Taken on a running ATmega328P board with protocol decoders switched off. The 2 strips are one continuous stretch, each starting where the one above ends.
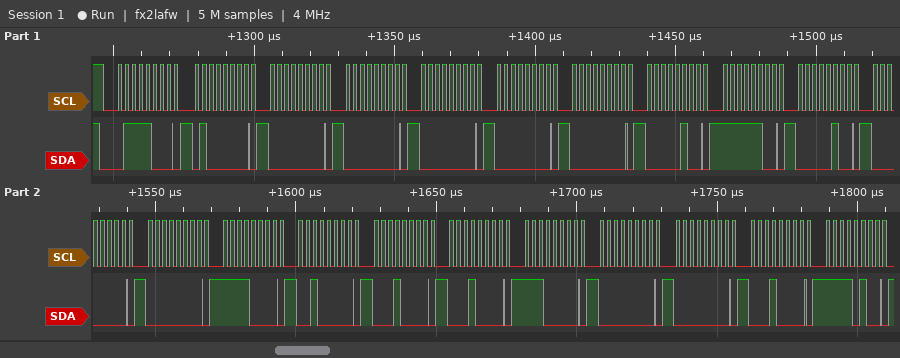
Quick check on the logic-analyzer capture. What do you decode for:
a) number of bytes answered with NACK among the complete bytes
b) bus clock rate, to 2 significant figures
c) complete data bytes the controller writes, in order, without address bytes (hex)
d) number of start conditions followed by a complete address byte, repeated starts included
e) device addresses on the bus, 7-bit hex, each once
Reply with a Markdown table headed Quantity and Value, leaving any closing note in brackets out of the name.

| Quantity | Value |
|---|---|
| number of bytes answered with NACK among the complete bytes | 0 |
| bus clock rate, to 2 significant figures | 400 kHz |
| complete data bytes the controller writes, in order, without address bytes | 40 00 00 00 00 00 04 FC 04 00 00 F0 20 10 10 E0 00 00 10 F4 |
| number of start conditions followed by a complete address byte, repeated starts included | 1 |
| device addresses on the bus, 7-bit hex, each once | 0x3C |
